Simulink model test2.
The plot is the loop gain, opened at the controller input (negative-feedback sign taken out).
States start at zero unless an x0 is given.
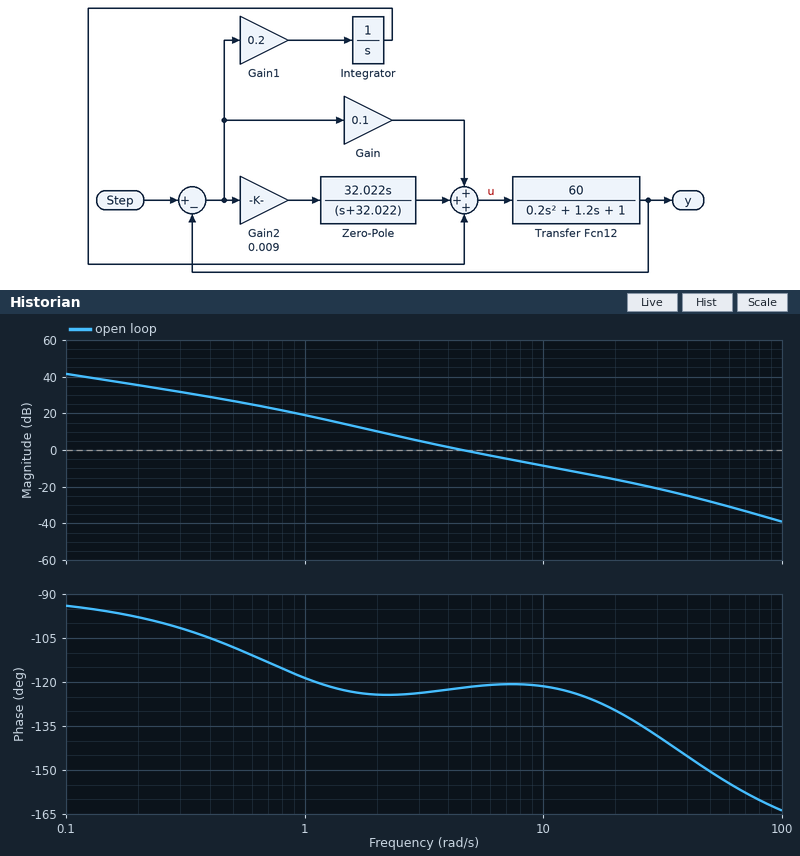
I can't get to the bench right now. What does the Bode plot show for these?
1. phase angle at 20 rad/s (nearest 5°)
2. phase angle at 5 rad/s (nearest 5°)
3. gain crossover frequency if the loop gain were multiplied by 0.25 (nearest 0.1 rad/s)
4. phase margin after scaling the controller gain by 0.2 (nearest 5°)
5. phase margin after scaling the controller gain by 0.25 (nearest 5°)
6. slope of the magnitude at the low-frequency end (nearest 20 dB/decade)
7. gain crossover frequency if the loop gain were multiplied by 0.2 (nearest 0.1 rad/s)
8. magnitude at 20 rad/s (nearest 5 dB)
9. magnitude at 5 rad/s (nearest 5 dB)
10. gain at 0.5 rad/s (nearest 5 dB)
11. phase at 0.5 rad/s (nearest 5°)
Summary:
-130°
-120°
1.7 rad/s
55°
55°
-20 dB/decade
1.5 rad/s
-15 dB
0 dB
25 dB
-110°
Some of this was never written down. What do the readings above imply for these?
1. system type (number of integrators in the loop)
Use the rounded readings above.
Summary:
1
